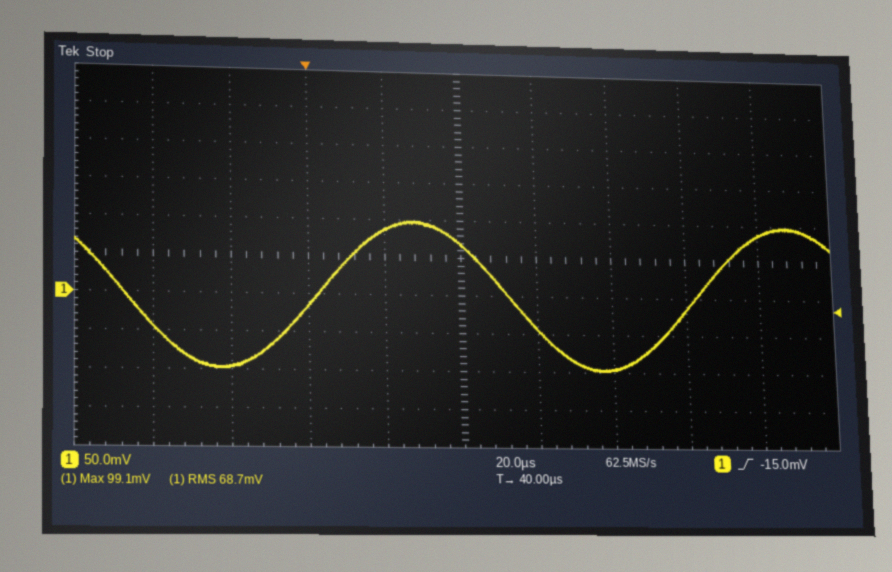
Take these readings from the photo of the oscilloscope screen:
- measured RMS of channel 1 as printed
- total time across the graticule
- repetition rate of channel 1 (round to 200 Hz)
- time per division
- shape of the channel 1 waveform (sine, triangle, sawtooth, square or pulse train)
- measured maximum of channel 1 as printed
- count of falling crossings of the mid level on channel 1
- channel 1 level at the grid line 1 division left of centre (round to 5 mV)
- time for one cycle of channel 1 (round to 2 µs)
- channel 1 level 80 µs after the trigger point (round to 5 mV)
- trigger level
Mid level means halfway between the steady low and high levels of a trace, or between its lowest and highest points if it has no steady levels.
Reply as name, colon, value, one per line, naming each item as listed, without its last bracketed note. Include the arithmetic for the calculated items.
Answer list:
measured RMS of channel 1 as printed: 68.7 mV
total time across the graticule: 200 µs
repetition rate of channel 1: 1 / 100 µs ≈ 10.0 kHz
time per division: 20 µs
shape of the channel 1 waveform: sine
measured maximum of channel 1 as printed: 99.1 mV
count of falling crossings of the mid level on channel 1: 2
channel 1 level at the grid line 1 division left of centre: 85 mV
time for one cycle of channel 1: 100 µs
channel 1 level 80 µs after the trigger point: -95 mV
trigger level: -15.0 mV
